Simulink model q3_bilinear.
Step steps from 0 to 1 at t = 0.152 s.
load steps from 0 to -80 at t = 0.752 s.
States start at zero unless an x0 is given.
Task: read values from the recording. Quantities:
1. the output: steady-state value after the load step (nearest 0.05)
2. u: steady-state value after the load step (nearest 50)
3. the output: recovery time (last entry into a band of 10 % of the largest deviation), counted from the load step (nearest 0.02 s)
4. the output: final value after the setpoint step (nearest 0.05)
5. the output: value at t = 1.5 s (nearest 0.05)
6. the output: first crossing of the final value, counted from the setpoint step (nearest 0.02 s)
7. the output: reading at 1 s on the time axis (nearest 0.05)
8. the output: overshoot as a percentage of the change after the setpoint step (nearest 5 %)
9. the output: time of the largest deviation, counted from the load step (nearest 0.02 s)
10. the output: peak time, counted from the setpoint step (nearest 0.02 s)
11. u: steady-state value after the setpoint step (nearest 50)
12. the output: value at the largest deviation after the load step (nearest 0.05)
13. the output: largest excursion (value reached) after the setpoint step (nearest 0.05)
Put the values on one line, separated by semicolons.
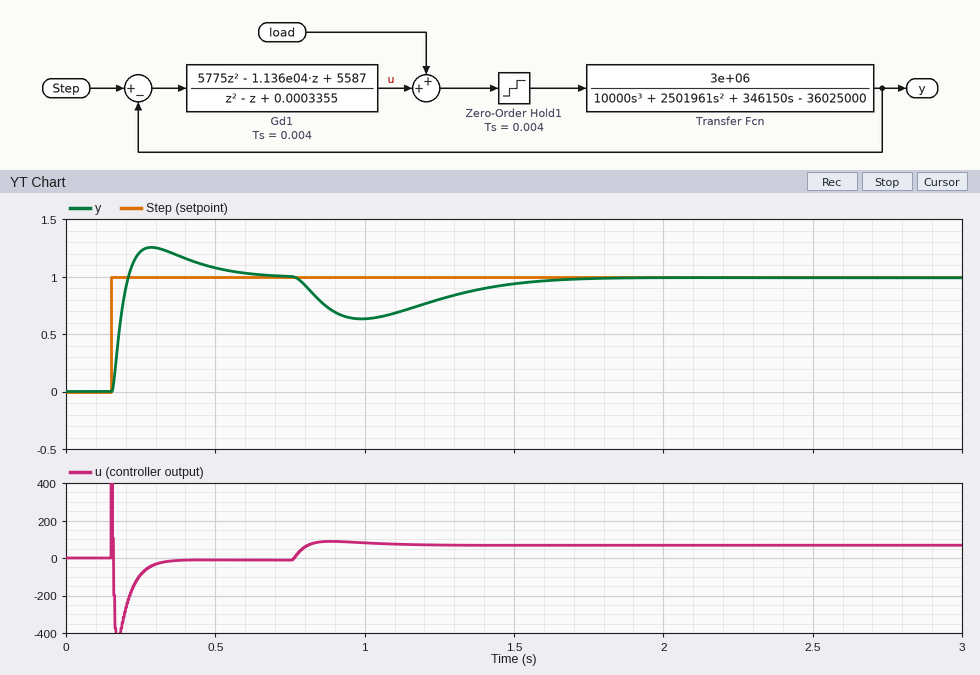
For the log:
1.00; 50; 0.80 s; 1.00; 0.95; 0.06 s; 0.65; 25 %; 0.24 s; 0.14 s; 0; 0.65; 1.25
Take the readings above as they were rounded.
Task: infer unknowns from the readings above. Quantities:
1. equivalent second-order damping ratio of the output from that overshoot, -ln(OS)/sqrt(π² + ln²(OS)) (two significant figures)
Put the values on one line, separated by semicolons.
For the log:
0.40
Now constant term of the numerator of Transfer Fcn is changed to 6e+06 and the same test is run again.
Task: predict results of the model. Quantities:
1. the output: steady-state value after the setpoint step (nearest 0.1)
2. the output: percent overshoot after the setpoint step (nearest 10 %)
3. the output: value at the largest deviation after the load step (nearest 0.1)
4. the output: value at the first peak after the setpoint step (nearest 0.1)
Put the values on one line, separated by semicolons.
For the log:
1.0; 20 %; 0.7; 1.2
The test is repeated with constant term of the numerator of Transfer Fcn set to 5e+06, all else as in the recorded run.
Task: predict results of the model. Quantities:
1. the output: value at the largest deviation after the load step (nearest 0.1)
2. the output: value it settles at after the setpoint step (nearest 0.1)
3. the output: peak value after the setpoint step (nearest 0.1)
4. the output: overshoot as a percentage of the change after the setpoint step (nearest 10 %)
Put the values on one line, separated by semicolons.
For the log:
0.7; 1.0; 1.2; 20 %
